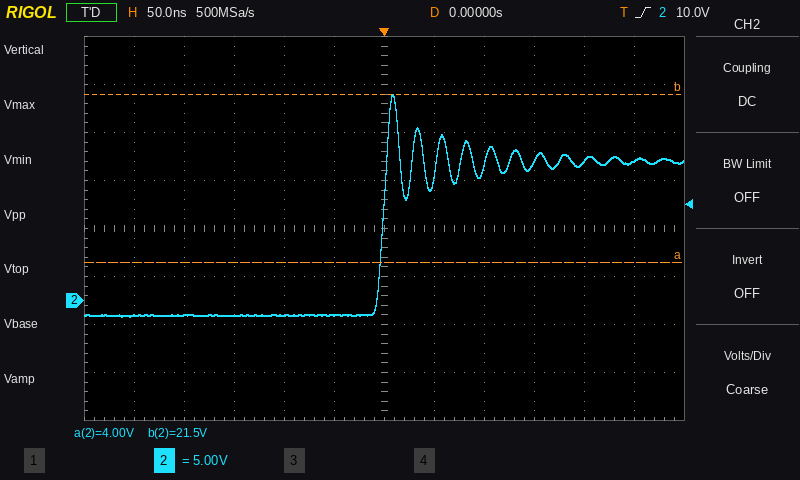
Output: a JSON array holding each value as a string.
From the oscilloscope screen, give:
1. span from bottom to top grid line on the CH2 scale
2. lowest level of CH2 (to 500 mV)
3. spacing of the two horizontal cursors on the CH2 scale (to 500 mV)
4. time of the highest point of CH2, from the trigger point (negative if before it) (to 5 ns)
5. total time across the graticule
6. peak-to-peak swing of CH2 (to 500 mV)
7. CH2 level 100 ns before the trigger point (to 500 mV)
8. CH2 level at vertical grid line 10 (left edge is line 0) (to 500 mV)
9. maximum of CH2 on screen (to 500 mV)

["40 V", "-1.5 V", "17.5 V", "+10 ns", "600 ns", "23.0 V", "-1.5 V", "14.5 V", "21.5 V"]
